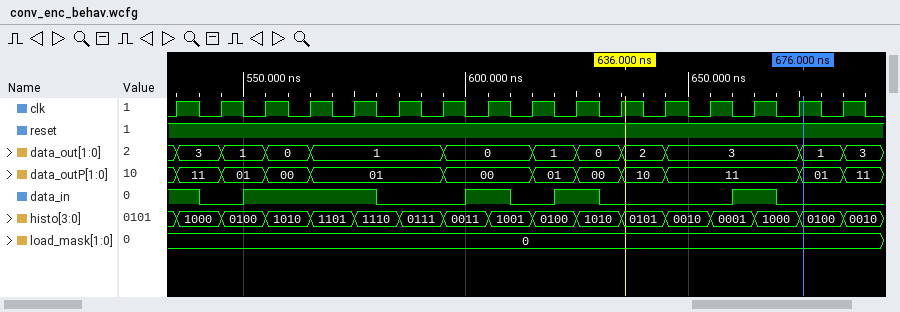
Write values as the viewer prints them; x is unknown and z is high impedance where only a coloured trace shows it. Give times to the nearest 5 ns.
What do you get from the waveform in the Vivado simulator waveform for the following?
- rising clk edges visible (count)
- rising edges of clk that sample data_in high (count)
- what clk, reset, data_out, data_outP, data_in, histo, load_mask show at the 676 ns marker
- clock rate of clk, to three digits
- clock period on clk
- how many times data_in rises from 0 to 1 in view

16
7
clk=1, reset=1, data_out=1, data_outP=01, data_in=0, histo=0100, load_mask=0
100 MHz
10 ns
4
